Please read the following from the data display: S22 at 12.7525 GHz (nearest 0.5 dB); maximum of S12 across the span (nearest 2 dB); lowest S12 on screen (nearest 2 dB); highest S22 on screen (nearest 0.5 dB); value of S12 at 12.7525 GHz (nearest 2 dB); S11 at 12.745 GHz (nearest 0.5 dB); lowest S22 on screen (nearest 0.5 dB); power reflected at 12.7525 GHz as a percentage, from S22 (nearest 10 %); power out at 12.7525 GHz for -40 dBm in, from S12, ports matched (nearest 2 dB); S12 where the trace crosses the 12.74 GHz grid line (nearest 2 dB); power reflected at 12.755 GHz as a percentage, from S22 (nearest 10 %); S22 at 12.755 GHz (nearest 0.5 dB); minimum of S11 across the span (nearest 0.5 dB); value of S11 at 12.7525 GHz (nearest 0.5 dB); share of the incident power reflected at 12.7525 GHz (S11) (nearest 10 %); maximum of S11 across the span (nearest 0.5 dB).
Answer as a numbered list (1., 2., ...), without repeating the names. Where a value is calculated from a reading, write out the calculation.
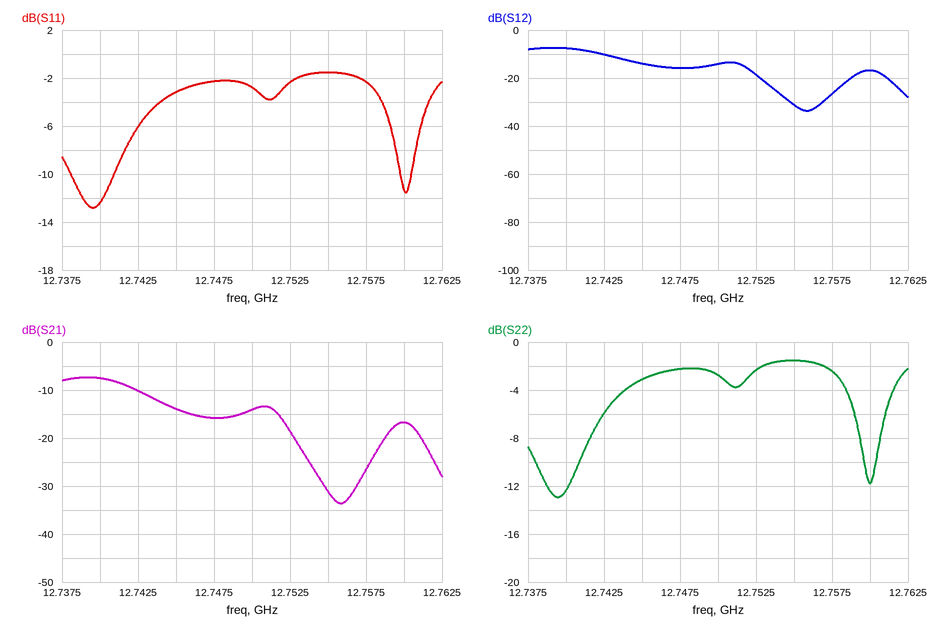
1. -2.5 dB
2. -8 dB
3. -34 dB
4. -1.5 dB
5. -18 dB
6. -3.0 dB
7. -13.0 dB
8. 10^(-2.5/10) ≈ 56.2 %, so 60 % to the nearest 10 %
9. -40 dBm + (-18 dB) = -58 dBm
10. -8 dB
11. 10^(-1.5/10) ≈ 70.8 %, so 70 % to the nearest 10 %
12. -1.5 dB
13. -13.0 dB
14. -2.5 dB
15. 10^(-2.5/10) ≈ 56.2 %, so 60 % to the nearest 10 %
16. -1.5 dB
